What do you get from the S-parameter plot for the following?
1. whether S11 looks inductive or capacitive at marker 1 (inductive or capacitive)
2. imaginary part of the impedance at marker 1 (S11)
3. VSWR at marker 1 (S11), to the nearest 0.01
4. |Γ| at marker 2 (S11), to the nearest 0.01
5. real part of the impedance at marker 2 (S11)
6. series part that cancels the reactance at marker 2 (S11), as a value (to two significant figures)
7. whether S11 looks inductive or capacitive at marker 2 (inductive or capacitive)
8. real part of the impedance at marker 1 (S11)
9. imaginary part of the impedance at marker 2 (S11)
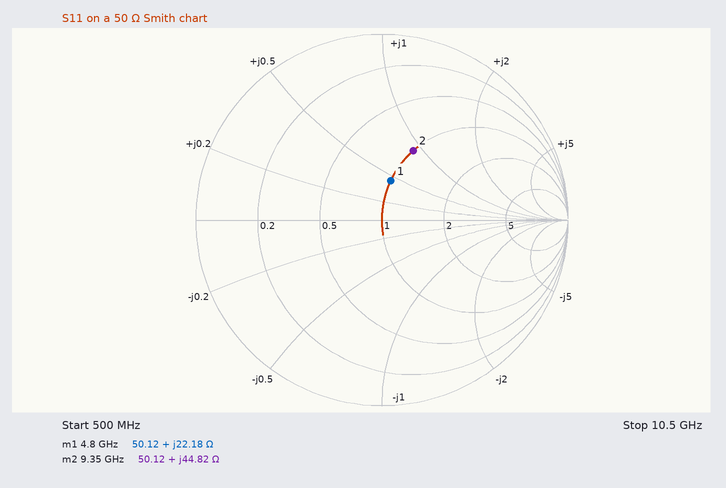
inductive
+22.18 Ω
1.55
0.41
50.12 Ω
380 fF
inductive
50.12 Ω
+44.82 Ω
